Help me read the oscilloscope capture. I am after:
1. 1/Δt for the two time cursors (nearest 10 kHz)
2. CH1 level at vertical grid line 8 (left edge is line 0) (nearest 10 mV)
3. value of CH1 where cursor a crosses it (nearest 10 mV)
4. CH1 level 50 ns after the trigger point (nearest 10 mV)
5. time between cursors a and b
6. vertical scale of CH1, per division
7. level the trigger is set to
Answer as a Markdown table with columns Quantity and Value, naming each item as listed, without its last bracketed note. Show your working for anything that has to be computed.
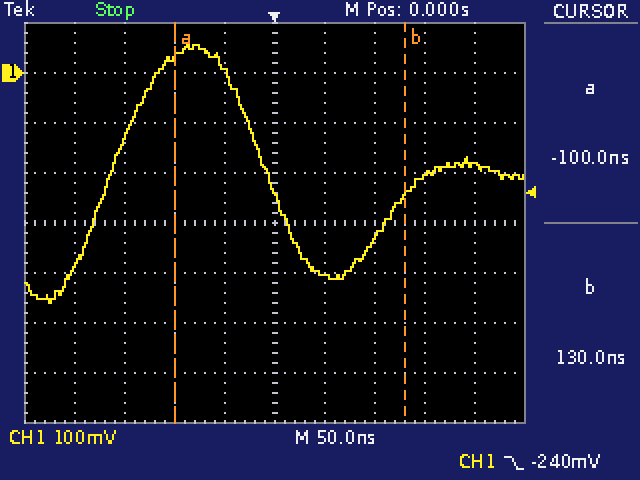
| Quantity | Value |
|---|---|
| 1/Δt for the two time cursors | 1 / 230 ns ≈ 4.35 MHz |
| CH1 level at vertical grid line 8 (left edge is line 0) | -200 mV |
| value of CH1 where cursor a crosses it | 30 mV |
| CH1 level 50 ns after the trigger point | -400 mV |
| time between cursors a and b | 130 ns − (-100 ns) = 230 ns |
| vertical scale of CH1, per division | 100 mV |
| level the trigger is set to | -240 mV |
